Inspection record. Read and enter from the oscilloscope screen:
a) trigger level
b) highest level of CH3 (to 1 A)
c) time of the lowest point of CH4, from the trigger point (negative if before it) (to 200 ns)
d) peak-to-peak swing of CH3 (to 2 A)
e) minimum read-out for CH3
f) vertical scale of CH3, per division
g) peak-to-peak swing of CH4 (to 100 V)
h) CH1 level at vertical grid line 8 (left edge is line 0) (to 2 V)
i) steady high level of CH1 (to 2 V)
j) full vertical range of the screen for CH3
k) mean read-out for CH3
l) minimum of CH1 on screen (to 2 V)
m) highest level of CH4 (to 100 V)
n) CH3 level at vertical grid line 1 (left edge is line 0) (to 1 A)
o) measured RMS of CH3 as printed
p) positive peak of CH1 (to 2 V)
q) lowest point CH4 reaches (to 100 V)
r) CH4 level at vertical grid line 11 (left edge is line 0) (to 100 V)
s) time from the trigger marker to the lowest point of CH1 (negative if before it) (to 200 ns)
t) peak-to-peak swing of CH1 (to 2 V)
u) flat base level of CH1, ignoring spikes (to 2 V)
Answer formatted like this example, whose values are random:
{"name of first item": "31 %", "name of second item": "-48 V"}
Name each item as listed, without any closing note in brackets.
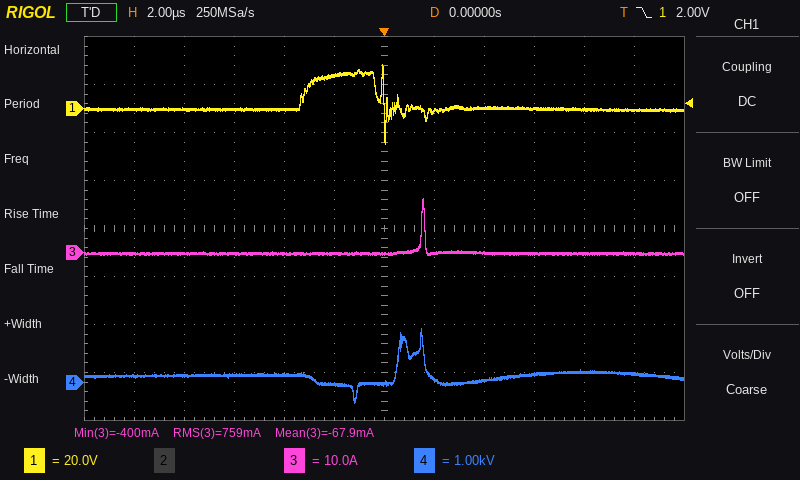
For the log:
{"trigger level": "2.00 V", "highest level of CH3": "11 A", "time of the lowest point of CH4, from the trigger point (negative if before it)": "-1.2 µs", "peak-to-peak swing of CH3": "12 A", "minimum read-out for CH3": "-400 mA", "vertical scale of CH3, per division": "10 A", "peak-to-peak swing of CH4": "1.5 kV", "CH1 level at vertical grid line 8 (left edge is line 0)": "0 V", "steady high level of CH1": "14 V", "full vertical range of the screen for CH3": "80 A", "mean read-out for CH3": "-67.9 mA", "minimum of CH1 on screen": "-14 V", "highest level of CH4": "1.1 kV", "CH3 level at vertical grid line 1 (left edge is line 0)": "0 A", "measured RMS of CH3 as printed": "759 mA", "positive peak of CH1": "18 V", "lowest point CH4 reaches": "-400 V", "CH4 level at vertical grid line 11 (left edge is line 0)": "200 V", "time from the trigger marker to the lowest point of CH1 (negative if before it)": "0.0 µs", "peak-to-peak swing of CH1": "32 V", "flat base level of CH1, ignoring spikes": "0 V"}
